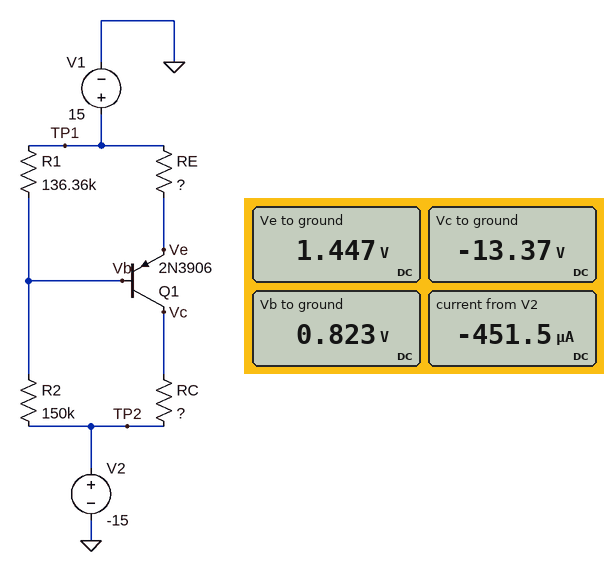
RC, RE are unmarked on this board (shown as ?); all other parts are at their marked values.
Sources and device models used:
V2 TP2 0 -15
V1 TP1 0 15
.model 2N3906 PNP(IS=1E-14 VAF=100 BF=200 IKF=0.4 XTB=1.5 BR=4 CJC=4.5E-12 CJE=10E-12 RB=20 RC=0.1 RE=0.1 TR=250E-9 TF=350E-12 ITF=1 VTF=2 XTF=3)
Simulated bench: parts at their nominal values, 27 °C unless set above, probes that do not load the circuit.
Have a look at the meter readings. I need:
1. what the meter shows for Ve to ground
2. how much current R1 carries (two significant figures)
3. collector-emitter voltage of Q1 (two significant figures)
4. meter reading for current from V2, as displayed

1.447 V
100 µA
-15 V
-451.5 µA
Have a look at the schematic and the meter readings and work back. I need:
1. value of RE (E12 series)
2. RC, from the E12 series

39 kΩ
4.7 kΩ
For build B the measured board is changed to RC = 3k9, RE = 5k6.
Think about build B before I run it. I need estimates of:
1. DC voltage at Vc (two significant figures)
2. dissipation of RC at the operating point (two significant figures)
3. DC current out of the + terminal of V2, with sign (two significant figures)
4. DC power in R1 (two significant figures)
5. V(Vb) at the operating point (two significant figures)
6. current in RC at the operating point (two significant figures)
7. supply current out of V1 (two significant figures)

-6.1 V
20 mW
-2.4 mA
1.3 mW
1.5 V
2.3 mA
2.4 mA
